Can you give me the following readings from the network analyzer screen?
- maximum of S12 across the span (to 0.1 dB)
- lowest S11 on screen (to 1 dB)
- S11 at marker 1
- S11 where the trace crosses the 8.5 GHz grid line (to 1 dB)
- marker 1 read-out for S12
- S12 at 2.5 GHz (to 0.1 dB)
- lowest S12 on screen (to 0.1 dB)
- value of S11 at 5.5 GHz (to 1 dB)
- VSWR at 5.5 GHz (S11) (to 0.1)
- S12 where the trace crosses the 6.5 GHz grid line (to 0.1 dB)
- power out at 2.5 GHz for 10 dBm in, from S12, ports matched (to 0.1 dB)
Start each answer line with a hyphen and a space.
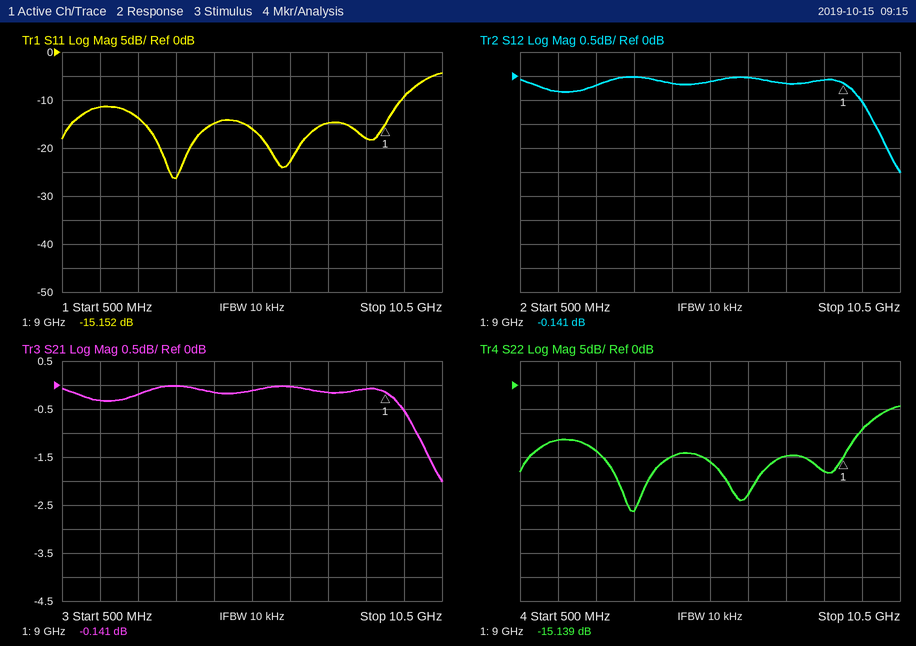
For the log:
- 0.0 dB
- -26 dB
- -15.152 dB
- -18 dB
- -0.141 dB
- -0.2 dB
- -2.0 dB
- -16 dB
- 1.4
- 0.0 dB
- 9.8 dBm
